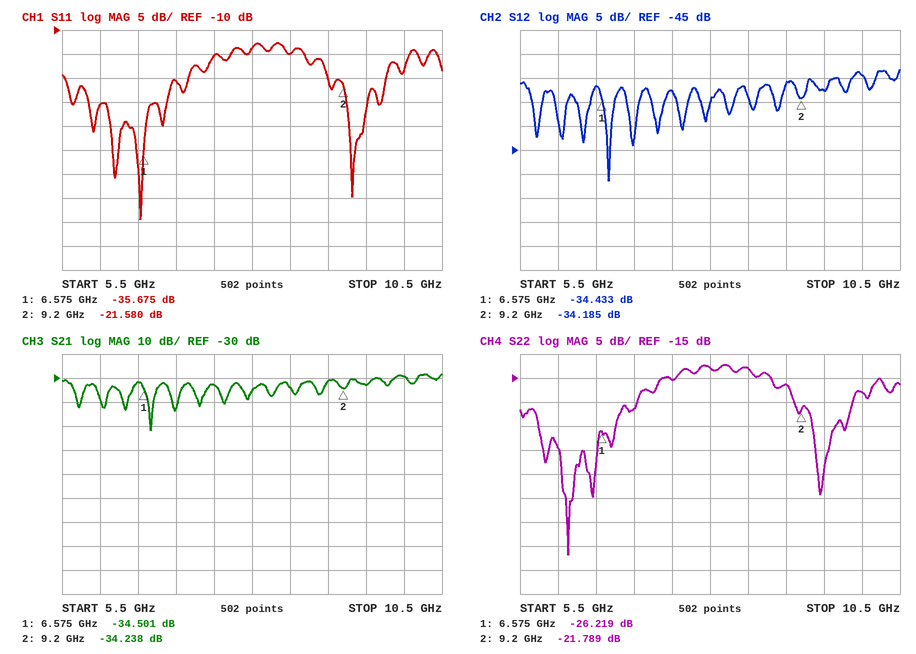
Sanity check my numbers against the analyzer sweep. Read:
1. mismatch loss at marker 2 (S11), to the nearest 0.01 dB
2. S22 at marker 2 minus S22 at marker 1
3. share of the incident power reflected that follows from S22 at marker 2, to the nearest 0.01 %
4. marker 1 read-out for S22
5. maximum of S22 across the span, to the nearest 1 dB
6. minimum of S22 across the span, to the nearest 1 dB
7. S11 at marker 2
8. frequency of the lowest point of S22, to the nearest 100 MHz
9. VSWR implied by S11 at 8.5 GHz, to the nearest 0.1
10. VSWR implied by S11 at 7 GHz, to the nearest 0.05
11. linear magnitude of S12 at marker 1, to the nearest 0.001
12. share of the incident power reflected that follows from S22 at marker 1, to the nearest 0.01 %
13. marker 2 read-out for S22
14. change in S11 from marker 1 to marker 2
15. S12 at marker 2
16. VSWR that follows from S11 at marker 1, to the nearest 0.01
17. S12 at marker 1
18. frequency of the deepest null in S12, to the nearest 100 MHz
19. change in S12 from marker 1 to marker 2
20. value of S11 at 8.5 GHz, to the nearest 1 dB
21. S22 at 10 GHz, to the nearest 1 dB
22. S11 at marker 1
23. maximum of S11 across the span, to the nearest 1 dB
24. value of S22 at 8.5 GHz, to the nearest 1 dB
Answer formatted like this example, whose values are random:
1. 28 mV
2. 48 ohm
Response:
1. 0.03 dB
2. 4.430 dB
3. 0.66 %
4. -26.219 dB
5. -12 dB
6. -52 dB
7. -21.580 dB
8. 6.1 GHz
9. 1.4
10. 1.20
11. 0.019
12. 0.24 %
13. -21.789 dB
14. 14.095 dB
15. -34.185 dB
16. 1.03
17. -34.433 dB
18. 6.7 GHz
19. 0.248 dB
20. -15 dB
21. -18 dB
22. -35.675 dB
23. -13 dB
24. -13 dB
